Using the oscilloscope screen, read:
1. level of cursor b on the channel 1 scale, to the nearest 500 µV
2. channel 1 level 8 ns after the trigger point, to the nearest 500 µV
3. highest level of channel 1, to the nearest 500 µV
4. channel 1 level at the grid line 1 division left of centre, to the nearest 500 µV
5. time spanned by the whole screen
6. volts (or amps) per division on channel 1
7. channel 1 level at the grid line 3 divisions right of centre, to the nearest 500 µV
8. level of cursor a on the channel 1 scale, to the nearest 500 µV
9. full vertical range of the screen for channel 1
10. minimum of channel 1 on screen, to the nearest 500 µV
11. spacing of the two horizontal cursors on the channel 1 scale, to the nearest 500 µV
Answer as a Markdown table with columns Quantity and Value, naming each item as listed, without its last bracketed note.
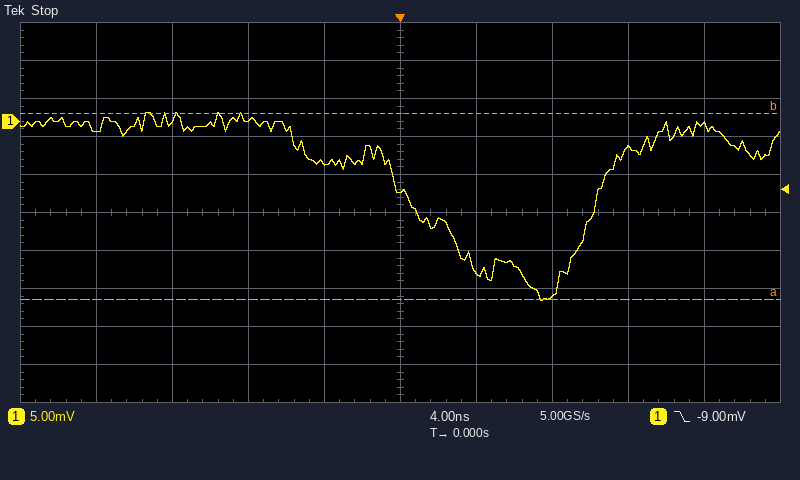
| Quantity | Value |
|---|---|
| level of cursor b on the channel 1 scale, to the nearest 500 µV | 1.0 mV |
| channel 1 level 8 ns after the trigger point, to the nearest 500 µV | -23.0 mV |
| highest level of channel 1, to the nearest 500 µV | 1.0 mV |
| channel 1 level at the grid line 1 division left of centre, to the nearest 500 µV | -5.5 mV |
| time spanned by the whole screen | 40 ns |
| volts (or amps) per division on channel 1 | 5 mV |
| channel 1 level at the grid line 3 divisions right of centre, to the nearest 500 µV | -3.5 mV |
| level of cursor a on the channel 1 scale, to the nearest 500 µV | -23.5 mV |
| full vertical range of the screen for channel 1 | 50 mV |
| minimum of channel 1 on screen, to the nearest 500 µV | -23.5 mV |
| spacing of the two horizontal cursors on the channel 1 scale, to the nearest 500 µV | 24.5 mV |
